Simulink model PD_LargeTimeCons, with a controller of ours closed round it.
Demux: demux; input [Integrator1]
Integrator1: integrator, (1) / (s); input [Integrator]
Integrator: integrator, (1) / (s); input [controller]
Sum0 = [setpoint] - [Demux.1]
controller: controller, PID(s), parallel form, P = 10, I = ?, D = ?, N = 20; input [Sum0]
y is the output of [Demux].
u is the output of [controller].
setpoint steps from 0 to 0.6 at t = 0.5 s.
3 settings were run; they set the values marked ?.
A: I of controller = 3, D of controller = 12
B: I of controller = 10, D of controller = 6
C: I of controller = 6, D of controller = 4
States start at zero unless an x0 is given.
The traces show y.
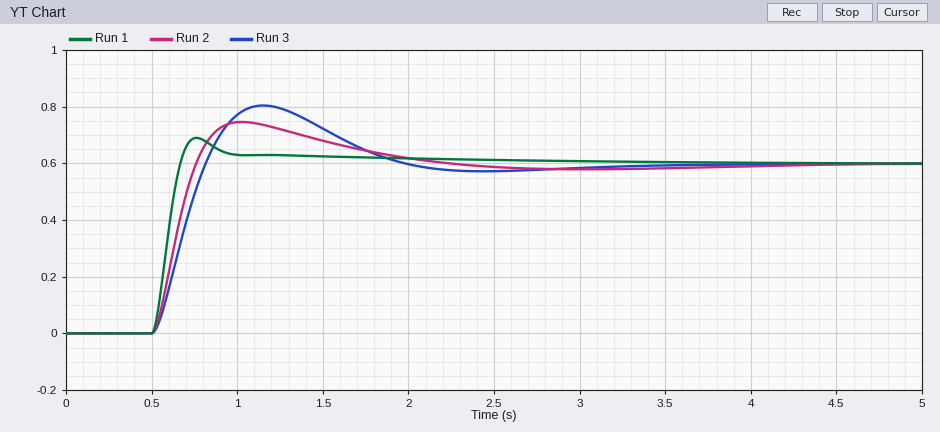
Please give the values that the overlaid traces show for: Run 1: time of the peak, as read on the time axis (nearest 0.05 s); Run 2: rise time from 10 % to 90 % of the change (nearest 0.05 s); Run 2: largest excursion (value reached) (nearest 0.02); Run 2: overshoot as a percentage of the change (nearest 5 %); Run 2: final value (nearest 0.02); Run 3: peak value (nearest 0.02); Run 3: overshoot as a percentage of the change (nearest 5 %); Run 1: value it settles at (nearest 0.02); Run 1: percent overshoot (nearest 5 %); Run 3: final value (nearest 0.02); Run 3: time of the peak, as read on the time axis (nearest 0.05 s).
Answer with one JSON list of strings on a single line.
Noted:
["0.75 s", "0.20 s", "0.74", "25 %", "0.60", "0.80", "35 %", "0.60", "15 %", "0.60", "1.15 s"]
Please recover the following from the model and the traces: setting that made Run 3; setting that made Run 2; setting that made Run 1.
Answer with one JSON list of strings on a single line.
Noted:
["C", "B", "A"]
